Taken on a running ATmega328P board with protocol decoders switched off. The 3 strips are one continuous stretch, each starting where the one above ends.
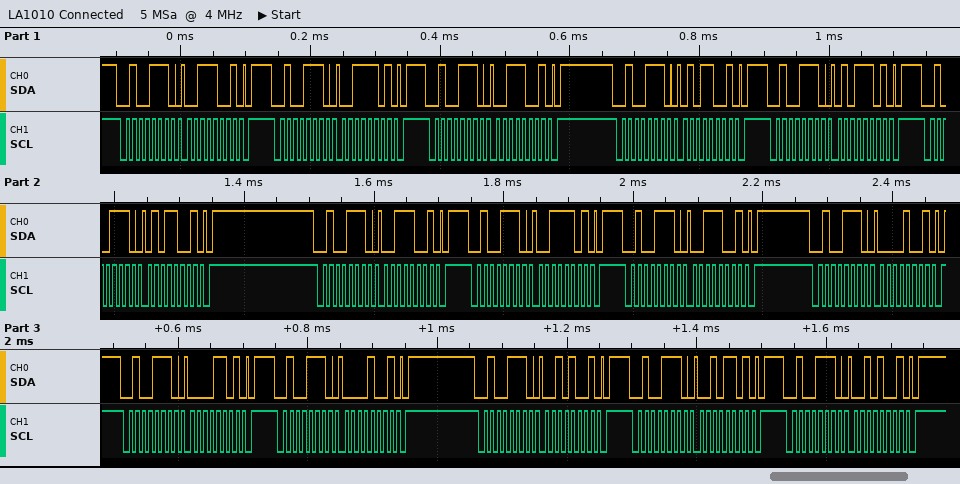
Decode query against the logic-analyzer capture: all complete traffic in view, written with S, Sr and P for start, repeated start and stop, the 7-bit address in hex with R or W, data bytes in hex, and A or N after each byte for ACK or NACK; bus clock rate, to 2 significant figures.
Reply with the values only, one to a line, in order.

S 27W A 39 A P S 27W A 3D A P S 27W A 39 A P S 27W A 59 A P S 27W A 5D A P S 27W A 59 A P S 27W A 39 A P S 27W A 3D A P S 27W A 39 A P S 27W A 09 A P S 27W A 0D A P S 27W A 09 A P S 27W A 29 A P S 27W A 2D A P S 27W A 29 A P
100 kHz
